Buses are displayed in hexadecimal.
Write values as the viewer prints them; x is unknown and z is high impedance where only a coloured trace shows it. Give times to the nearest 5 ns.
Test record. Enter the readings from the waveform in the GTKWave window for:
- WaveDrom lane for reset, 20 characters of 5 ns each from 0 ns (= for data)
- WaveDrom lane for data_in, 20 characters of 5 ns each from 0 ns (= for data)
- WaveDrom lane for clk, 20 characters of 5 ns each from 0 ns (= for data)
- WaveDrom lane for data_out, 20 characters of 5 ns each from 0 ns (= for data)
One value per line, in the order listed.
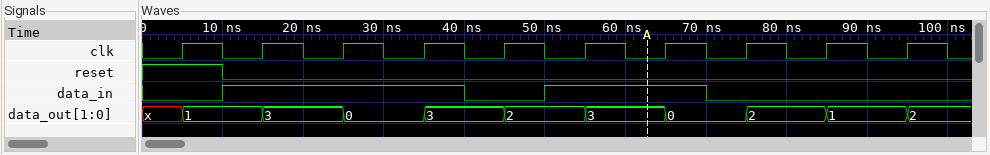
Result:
{name: 'reset', wave: '1.0.................'}
{name: 'data_in', wave: '0.1.....0.1...0.....'}
{name: 'clk', wave: '01010101010101010101'}
{name: 'data_out', wave: 'x=.=.=.=.=.=.=.=.=.=', data: '1 3 0 3 2 3 0 2 1 2'}
